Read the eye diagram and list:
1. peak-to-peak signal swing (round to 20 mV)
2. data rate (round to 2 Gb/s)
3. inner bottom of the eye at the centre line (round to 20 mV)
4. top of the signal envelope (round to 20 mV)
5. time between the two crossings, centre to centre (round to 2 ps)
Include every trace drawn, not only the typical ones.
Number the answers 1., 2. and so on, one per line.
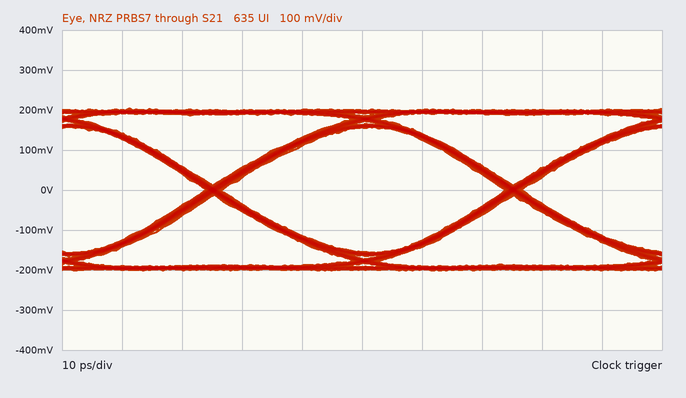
1. 400 mV
2. 20 Gb/s
3. -160 mV
4. 200 mV
5. 50 ps
